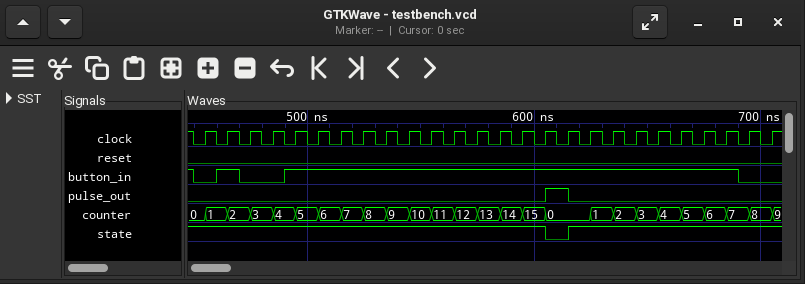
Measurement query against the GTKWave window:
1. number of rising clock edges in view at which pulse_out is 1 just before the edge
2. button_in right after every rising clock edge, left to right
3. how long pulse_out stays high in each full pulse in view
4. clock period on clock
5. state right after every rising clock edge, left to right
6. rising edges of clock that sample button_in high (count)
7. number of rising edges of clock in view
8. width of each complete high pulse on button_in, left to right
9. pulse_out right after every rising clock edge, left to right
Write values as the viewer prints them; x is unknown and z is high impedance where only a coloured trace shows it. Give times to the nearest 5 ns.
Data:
1
0 1 0 0 1 1 1 1 1 1 1 1 1 1 1 1 1 1 1 1 1 1 1 1 0 0
10 ns
10 ns
1 1 1 1 1 1 1 1 1 1 1 1 1 1 1 0 1 1 1 1 1 1 1 1 1 1
21
26
10 ns, 200 ns
0 0 0 0 0 0 0 0 0 0 0 0 0 0 0 1 0 0 0 0 0 0 0 0 0 0
